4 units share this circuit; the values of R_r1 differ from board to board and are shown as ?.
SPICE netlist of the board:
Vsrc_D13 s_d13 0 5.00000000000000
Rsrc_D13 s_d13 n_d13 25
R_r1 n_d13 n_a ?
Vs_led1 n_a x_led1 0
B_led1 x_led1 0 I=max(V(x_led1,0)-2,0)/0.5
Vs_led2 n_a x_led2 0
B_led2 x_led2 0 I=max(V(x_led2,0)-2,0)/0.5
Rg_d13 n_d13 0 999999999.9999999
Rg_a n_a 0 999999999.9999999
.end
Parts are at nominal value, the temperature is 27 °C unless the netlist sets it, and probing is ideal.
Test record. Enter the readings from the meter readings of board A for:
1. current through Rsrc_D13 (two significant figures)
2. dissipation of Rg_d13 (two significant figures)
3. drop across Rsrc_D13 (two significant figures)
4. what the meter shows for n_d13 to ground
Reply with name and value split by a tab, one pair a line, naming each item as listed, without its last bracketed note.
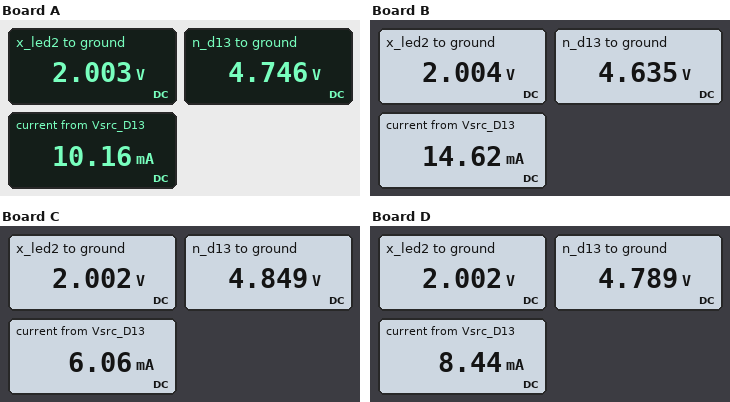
current through Rsrc_D13	10 mA
dissipation of Rg_d13	23 nW
drop across Rsrc_D13	250 mV
what the meter shows for n_d13 to ground	4.746 V
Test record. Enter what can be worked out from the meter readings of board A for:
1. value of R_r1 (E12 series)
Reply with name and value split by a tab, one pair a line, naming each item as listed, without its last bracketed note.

value of R_r1	270 Ω
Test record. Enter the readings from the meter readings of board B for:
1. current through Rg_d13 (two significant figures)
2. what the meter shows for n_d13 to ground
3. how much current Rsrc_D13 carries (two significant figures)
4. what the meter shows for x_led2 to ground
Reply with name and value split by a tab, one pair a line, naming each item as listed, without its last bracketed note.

current through Rg_d13	4.6 nA
what the meter shows for n_d13 to ground	4.635 V
how much current Rsrc_D13 carries	15 mA
what the meter shows for x_led2 to ground	2.004 V
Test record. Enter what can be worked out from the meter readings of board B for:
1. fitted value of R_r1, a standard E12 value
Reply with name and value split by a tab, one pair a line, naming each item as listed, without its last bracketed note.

fitted value of R_r1, a standard E12 value	180 Ω
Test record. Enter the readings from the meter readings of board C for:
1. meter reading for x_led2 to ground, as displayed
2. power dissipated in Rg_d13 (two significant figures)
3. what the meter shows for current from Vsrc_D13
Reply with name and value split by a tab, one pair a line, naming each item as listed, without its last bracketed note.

meter reading for x_led2 to ground, as displayed	2.002 V
power dissipated in Rg_d13	24 nW
what the meter shows for current from Vsrc_D13	6.06 mA
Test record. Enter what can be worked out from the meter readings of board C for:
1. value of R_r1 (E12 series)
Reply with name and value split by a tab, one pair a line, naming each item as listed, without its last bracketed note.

value of R_r1	470 Ω
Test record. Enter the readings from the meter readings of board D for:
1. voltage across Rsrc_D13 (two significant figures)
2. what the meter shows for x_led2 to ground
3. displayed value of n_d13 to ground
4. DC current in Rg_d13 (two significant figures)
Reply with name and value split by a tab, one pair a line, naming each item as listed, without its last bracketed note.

voltage across Rsrc_D13	210 mV
what the meter shows for x_led2 to ground	2.002 V
displayed value of n_d13 to ground	4.789 V
DC current in Rg_d13	4.8 nA
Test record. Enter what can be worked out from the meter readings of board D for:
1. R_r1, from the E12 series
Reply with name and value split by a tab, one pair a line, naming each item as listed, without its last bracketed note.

R_r1, from the E12 series	330 Ω
